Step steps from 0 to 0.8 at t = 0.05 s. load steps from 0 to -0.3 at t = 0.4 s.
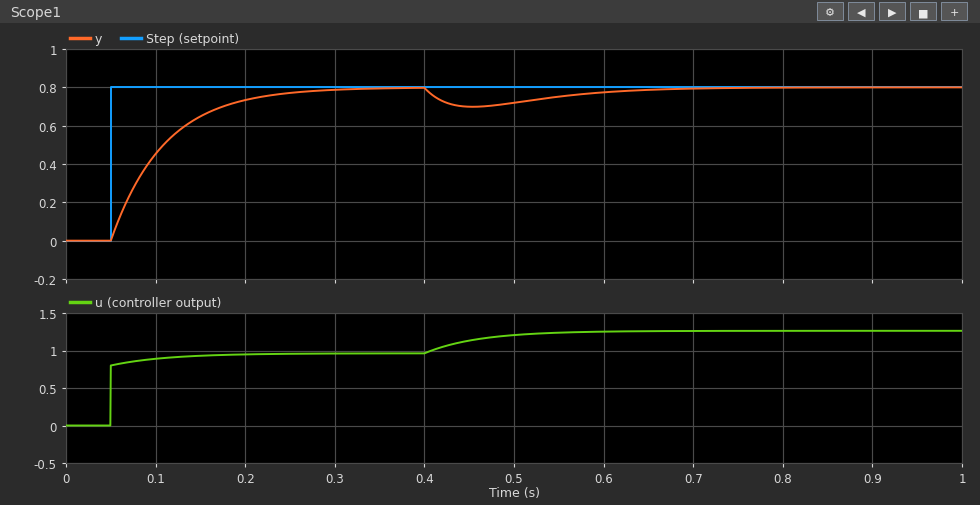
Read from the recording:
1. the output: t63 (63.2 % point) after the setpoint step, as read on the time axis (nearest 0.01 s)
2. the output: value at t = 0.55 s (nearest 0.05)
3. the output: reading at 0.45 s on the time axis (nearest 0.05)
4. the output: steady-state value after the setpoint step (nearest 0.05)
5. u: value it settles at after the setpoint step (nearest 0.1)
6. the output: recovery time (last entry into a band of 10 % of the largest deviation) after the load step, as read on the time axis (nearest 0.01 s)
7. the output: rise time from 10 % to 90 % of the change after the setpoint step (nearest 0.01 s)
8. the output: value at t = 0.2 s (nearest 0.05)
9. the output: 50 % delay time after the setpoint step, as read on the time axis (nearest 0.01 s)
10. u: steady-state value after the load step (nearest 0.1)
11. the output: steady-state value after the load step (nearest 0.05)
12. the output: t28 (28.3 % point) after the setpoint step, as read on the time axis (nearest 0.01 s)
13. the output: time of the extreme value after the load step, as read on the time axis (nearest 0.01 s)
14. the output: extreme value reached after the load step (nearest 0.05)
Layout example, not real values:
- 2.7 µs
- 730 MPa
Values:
- 0.11 s
- 0.75
- 0.70
- 0.80
- 1.0
- 0.67 s
- 0.13 s
- 0.75
- 0.09 s
- 1.3
- 0.80
- 0.07 s
- 0.45 s
- 0.70
